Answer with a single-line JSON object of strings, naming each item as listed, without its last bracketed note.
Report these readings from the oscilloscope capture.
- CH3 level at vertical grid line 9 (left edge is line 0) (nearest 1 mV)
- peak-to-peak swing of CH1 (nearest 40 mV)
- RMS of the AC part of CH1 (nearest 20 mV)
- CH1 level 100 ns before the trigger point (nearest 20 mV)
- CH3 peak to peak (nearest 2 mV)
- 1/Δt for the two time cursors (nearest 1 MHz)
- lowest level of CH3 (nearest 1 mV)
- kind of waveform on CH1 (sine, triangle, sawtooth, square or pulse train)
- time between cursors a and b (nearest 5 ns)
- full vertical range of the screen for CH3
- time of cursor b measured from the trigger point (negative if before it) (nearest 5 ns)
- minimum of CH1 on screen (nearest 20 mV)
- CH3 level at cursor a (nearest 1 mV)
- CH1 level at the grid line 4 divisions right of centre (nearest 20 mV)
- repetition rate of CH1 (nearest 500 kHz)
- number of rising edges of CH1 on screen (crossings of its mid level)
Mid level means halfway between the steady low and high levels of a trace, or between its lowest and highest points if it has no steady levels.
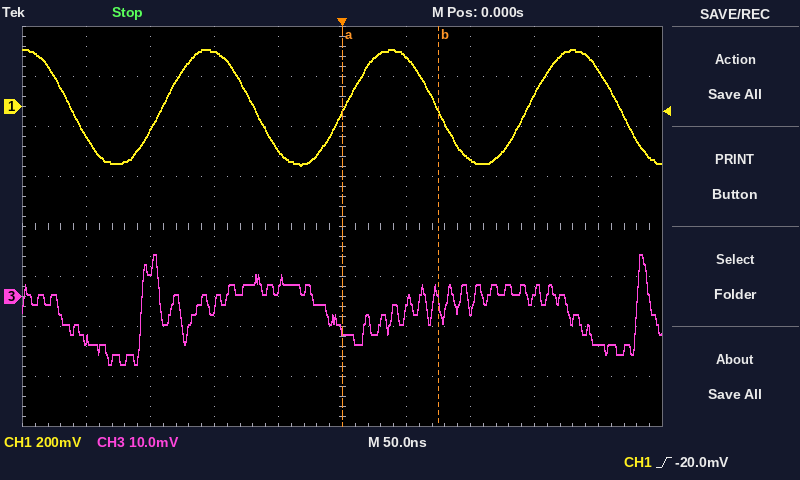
{"CH3 level at vertical grid line 9 (left edge is line 0)": "-10 mV", "peak-to-peak swing of CH1": "480 mV", "RMS of the AC part of CH1": "160 mV", "CH1 level 100 ns before the trigger point": "220 mV", "CH3 peak to peak": "22 mV", "1/Δt for the two time cursors": "13 MHz", "lowest level of CH3": "-14 mV", "kind of waveform on CH1": "sine", "time between cursors a and b": "75 ns", "full vertical range of the screen for CH3": "80 mV", "time of cursor b measured from the trigger point (negative if before it)": "+75 ns", "minimum of CH1 on screen": "-240 mV", "CH3 level at cursor a": "-7 mV", "CH1 level at the grid line 4 divisions right of centre": "140 mV", "repetition rate of CH1": "7.0 MHz", "number of rising edges of CH1 on screen": "3"}
